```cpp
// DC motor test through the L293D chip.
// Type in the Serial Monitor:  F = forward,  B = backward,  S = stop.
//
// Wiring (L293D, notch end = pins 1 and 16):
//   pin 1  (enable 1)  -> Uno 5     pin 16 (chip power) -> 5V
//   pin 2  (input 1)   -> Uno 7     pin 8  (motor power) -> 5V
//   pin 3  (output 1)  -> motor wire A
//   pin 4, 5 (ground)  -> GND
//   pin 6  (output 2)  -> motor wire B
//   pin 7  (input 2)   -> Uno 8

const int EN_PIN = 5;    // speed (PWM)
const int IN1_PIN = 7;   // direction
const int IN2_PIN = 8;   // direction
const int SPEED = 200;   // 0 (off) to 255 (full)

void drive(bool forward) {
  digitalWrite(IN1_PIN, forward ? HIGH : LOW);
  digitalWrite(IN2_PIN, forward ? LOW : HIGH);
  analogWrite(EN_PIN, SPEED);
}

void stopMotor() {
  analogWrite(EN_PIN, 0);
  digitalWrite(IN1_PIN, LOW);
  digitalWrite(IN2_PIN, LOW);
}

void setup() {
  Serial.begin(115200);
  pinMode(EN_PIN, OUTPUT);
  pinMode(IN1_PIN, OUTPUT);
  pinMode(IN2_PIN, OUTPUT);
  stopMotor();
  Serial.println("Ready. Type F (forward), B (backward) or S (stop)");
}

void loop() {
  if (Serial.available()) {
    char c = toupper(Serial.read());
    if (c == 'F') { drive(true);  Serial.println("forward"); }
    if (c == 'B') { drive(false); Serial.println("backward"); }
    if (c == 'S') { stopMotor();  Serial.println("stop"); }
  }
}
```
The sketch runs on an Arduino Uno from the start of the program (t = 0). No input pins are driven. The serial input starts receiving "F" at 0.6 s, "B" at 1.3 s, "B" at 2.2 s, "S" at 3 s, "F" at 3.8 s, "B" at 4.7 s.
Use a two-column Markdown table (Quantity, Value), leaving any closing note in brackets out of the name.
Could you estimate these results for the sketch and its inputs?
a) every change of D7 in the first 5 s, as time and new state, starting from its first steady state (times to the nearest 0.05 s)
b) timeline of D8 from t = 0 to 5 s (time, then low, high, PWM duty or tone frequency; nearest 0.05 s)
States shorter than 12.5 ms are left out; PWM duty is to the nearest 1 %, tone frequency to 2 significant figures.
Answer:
| Quantity | Value |
|---|---|
| every change of D7 in the first 5 s, as time and new state, starting from its first steady state | 0 s low; 0.6 s high; 1.3 s low; 3.8 s high; 4.7 s low |
| timeline of D8 from t = 0 to 5 s | 0 s low; 1.3 s high; 3 s low; 4.7 s high |
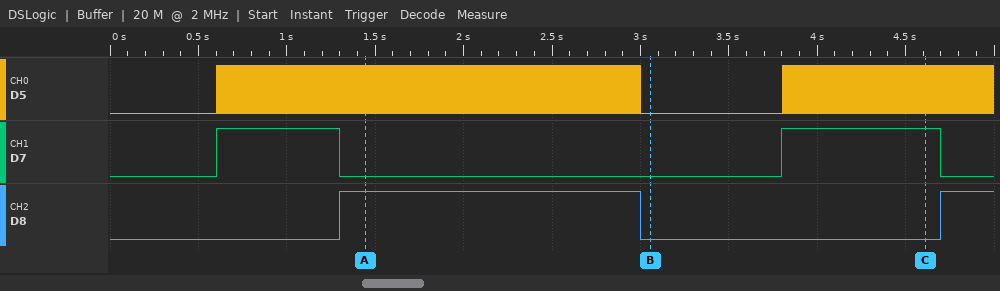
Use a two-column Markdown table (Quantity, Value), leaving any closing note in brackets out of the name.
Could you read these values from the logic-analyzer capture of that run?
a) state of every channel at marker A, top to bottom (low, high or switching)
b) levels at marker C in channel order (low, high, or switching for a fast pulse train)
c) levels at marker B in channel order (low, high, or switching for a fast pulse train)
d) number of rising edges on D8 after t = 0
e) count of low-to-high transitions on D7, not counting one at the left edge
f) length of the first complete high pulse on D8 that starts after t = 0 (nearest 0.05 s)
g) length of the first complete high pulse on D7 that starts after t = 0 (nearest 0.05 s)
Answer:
| Quantity | Value |
|---|---|
| state of every channel at marker A, top to bottom | D5 switching, D7 low, D8 high |
| levels at marker C in channel order | D5 switching, D7 high, D8 low |
| levels at marker B in channel order | D5 low, D7 low, D8 low |
| number of rising edges on D8 after t = 0 | 2 |
| count of low-to-high transitions on D7, not counting one at the left edge | 2 |
| length of the first complete high pulse on D8 that starts after t = 0 | 1.70 s |
| length of the first complete high pulse on D7 that starts after t = 0 | 0.70 s |
